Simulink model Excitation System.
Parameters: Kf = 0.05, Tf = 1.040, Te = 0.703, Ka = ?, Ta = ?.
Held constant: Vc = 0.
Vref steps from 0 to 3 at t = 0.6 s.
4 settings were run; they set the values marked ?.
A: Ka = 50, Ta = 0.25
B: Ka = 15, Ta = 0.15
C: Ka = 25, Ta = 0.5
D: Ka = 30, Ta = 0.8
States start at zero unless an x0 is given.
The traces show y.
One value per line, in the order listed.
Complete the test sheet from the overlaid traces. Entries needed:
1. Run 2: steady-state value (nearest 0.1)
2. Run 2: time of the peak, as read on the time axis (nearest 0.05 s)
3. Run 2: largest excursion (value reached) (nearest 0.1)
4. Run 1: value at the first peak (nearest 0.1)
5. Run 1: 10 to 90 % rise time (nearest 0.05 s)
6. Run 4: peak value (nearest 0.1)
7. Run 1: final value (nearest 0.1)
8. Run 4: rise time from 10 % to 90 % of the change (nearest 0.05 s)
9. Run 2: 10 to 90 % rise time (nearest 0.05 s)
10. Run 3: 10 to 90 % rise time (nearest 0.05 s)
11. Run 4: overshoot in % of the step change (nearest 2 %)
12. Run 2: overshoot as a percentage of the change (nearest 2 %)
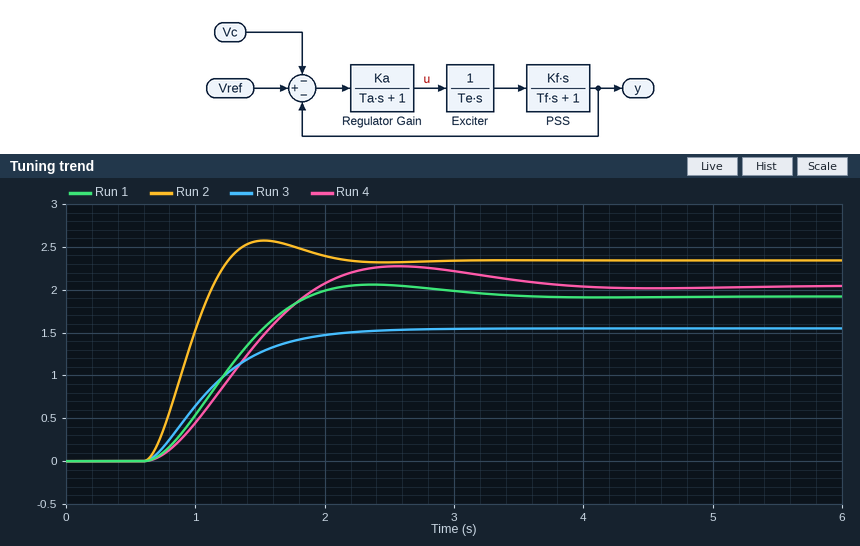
2.3
1.55 s
2.6
2.1
0.85 s
2.3
1.9
0.90 s
0.45 s
1.00 s
12 %
10 %
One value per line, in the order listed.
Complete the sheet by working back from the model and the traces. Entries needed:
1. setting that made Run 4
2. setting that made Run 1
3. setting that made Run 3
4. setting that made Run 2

D
C
B
A
